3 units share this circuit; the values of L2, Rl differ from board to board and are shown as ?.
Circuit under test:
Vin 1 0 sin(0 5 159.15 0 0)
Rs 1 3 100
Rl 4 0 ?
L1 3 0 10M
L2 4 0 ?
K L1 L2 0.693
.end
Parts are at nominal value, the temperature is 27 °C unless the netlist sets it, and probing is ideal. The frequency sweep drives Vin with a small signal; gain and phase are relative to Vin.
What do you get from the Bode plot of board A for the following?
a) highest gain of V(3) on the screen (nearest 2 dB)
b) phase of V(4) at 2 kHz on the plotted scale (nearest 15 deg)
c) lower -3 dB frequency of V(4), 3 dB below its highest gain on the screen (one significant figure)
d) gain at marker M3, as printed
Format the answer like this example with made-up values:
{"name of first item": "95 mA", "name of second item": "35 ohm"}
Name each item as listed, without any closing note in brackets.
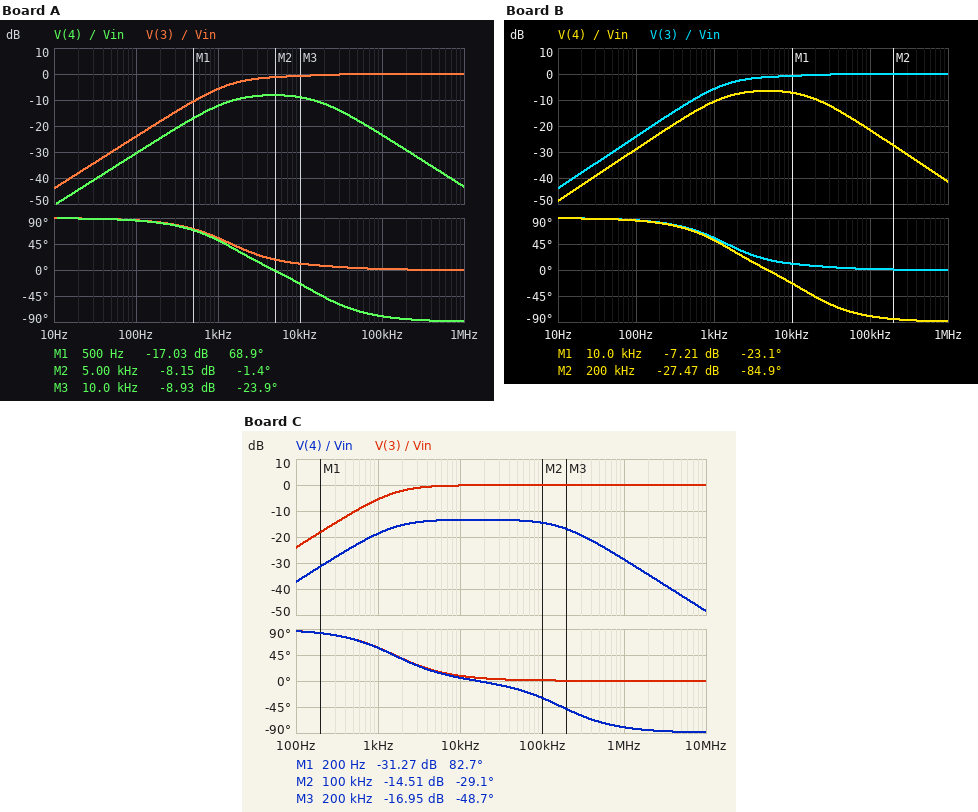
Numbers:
{"highest gain of V(3) on the screen": "0 dB", "phase of V(4) at 2 kHz on the plotted scale": "30 deg", "lower -3 dB frequency of V(4), 3 dB below its highest gain on the screen": "1 kHz", "gain at marker M3, as printed": "-8.93 dB"}
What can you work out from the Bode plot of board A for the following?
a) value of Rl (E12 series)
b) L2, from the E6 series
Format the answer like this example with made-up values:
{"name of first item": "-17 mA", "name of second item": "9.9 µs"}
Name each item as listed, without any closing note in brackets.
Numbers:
{"value of Rl": "220 Ω", "L2, from the E6 series": "4.7 mH"}
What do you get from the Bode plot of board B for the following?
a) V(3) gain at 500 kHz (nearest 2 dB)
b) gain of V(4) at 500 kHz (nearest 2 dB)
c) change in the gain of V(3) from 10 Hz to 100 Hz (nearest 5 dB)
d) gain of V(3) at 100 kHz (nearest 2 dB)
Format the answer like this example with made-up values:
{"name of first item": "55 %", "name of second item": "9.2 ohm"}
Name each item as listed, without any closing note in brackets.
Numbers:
{"V(3) gain at 500 kHz": "0 dB", "gain of V(4) at 500 kHz": "-36 dB", "change in the gain of V(3) from 10 Hz to 100 Hz": "20 dB", "gain of V(3) at 100 kHz": "0 dB"}
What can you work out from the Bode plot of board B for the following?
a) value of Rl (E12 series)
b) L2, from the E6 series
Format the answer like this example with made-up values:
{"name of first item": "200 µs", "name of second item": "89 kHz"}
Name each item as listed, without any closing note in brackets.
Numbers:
{"value of Rl": "330 Ω", "L2, from the E6 series": "6.8 mH"}
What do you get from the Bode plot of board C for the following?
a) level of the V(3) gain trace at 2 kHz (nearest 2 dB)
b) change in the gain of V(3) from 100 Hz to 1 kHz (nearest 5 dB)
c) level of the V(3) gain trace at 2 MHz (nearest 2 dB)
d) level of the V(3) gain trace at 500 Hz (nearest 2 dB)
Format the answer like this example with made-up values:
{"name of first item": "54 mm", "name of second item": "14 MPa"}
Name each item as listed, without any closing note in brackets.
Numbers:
{"level of the V(3) gain trace at 2 kHz": "-2 dB", "change in the gain of V(3) from 100 Hz to 1 kHz": "20 dB", "level of the V(3) gain trace at 2 MHz": "0 dB", "level of the V(3) gain trace at 500 Hz": "-10 dB"}
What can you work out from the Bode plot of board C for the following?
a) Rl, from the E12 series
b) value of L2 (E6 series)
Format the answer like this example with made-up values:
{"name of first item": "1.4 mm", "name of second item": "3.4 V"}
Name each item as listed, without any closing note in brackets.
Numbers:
{"Rl, from the E12 series": "560 Ω", "value of L2": "1 mH"}
